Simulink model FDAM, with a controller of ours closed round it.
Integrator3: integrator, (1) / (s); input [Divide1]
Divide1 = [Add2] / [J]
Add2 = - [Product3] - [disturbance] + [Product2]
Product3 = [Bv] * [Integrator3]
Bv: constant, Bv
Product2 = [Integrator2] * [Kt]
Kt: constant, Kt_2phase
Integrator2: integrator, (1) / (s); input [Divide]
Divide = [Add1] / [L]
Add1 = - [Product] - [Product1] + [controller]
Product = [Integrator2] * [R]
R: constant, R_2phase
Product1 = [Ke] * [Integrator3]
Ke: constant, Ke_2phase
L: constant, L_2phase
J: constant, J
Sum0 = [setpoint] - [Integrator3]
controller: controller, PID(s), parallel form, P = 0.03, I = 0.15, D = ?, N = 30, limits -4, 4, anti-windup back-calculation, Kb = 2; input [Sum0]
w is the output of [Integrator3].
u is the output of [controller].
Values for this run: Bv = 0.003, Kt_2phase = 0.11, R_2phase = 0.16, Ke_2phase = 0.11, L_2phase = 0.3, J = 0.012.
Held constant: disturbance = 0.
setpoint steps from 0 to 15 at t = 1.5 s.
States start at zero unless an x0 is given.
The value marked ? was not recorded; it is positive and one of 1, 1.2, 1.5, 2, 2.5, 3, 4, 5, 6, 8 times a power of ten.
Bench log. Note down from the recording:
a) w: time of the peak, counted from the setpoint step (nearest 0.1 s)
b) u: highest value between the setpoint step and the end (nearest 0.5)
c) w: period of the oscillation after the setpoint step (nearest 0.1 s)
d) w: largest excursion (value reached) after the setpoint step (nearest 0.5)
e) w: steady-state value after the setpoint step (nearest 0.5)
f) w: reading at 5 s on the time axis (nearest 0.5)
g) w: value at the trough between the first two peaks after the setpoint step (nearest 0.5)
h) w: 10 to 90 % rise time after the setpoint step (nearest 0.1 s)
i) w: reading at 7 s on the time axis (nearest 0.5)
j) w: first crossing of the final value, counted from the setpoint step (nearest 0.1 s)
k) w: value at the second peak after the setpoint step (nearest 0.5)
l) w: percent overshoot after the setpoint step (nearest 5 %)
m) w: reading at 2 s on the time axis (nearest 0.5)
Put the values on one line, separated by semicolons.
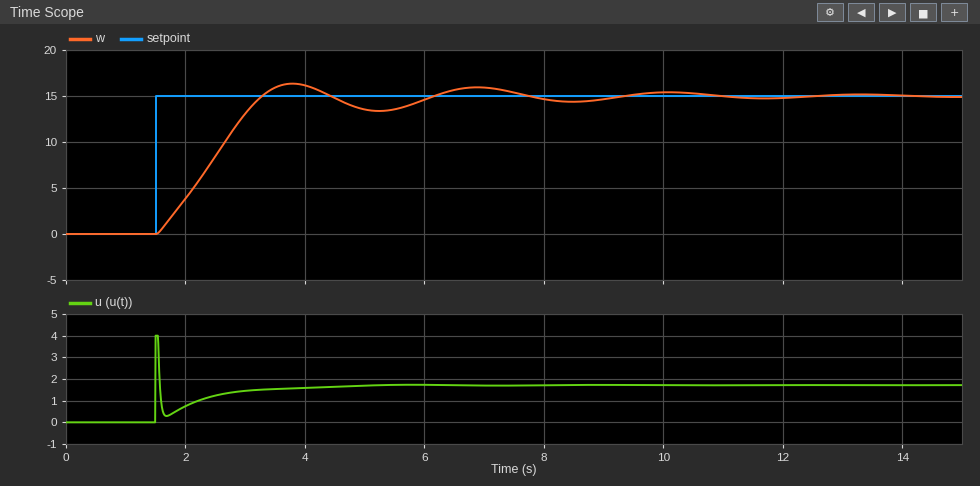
2.3 s; 4.0; 3.1 s; 16.5; 15.0; 13.5; 13.5; 1.3 s; 16.0; 1.8 s; 16.0; 10 %; 4.0
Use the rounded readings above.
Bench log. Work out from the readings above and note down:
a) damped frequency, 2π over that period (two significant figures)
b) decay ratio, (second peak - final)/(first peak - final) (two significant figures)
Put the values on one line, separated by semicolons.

2.0 rad/s; 0.67
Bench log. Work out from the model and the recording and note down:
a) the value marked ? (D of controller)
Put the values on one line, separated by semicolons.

0.03
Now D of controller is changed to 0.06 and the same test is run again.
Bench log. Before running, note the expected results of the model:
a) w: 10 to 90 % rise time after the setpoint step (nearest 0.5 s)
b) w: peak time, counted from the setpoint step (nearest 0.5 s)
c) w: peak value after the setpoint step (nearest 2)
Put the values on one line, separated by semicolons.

2.0 s; 3.0 s; 18
